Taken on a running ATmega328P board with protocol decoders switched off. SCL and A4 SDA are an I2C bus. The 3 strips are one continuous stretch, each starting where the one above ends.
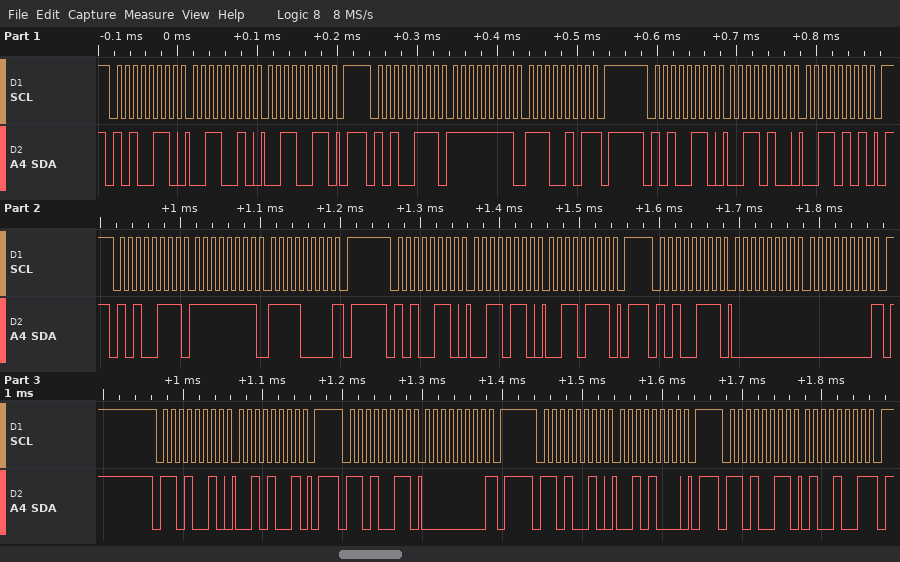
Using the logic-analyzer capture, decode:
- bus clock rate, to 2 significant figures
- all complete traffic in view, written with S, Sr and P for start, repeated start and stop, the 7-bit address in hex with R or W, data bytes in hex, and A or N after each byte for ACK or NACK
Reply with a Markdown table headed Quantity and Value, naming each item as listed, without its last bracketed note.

| Quantity | Value |
|---|---|
| bus clock rate, to 2 significant figures | 100 kHz |
| all complete traffic in view, written with S, Sr and P for start, repeated start and stop, the 7-bit address in hex with R or W, data bytes in hex, and A or N after each byte for ACK or NACK | S 53W A 32 A 33 A P S 53R A FF A E5 N P S 53W A 34 A 35 A P S 53R A FF A F0 N P S 53W A 36 A 37 A P S 53R A 00 A 00 N P S 69W A 29 A P S 69R A 00 N P S 69W A 28 A P S 69R A 49 N P |
